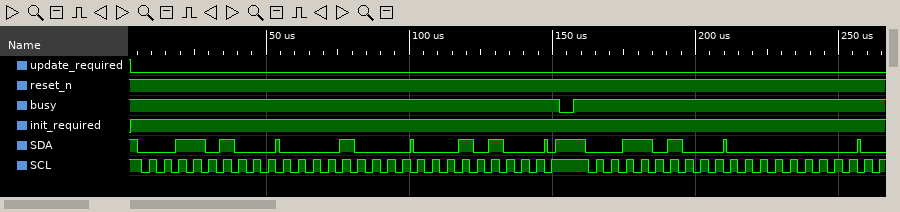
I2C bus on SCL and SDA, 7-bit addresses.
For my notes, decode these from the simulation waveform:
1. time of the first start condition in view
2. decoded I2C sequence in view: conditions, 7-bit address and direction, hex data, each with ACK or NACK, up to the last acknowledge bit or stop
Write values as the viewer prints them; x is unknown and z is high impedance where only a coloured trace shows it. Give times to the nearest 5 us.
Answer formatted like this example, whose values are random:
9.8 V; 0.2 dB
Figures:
5 us; start, address 1A write ACK, 08 ACK, 14 ACK, stop, start, address 1A write ACK, 00 ACK
